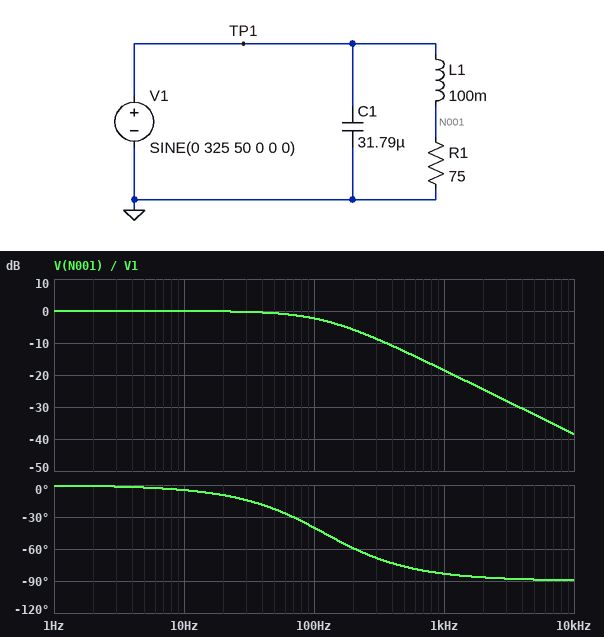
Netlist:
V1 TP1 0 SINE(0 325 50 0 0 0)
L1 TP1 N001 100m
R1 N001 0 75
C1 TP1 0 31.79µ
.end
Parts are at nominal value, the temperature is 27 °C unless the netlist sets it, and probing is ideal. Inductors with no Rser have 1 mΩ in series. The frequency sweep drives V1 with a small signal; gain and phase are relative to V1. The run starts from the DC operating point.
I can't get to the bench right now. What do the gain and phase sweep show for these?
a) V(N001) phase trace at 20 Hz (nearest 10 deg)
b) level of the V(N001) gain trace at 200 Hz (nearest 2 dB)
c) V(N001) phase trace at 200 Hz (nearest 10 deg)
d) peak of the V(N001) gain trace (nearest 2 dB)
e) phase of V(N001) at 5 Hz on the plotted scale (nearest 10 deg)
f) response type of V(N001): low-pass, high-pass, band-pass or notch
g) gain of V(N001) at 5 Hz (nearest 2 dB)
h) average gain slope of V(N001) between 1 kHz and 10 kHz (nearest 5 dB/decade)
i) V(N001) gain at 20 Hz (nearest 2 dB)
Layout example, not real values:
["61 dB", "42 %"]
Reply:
["-10 deg", "-6 dB", "-60 deg", "0 dB", "0 deg", "low-pass", "0 dB", "-20 dB/decade", "0 dB"]
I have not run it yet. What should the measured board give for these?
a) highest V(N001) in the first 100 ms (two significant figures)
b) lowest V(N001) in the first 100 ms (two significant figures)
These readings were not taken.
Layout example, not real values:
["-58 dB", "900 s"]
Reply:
["300 V", "-300 V"]
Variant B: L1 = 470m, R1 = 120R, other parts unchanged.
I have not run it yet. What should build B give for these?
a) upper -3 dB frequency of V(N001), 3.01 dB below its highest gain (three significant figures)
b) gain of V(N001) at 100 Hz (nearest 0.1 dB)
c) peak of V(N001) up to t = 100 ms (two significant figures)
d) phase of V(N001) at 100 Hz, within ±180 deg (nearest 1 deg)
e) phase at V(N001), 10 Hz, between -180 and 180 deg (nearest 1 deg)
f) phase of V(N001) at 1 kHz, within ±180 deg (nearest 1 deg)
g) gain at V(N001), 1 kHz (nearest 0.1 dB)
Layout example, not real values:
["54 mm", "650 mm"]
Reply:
["40.6 Hz", "-8.5 dB", "230 V", "-68 deg", "-14 deg", "-88 deg", "-27.8 dB"]
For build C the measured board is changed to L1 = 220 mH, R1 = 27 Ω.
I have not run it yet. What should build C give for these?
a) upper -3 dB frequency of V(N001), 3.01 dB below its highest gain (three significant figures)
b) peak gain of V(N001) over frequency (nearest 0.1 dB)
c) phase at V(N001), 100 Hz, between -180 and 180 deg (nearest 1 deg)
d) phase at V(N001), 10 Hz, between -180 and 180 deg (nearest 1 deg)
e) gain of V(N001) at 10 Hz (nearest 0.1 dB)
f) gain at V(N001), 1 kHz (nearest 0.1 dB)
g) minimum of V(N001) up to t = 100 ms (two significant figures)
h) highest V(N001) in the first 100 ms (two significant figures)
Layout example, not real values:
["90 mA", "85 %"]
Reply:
["19.5 Hz", "0 dB", "-79 deg", "-27 deg", "-1.0 dB", "-34.2 dB", "-120 V", "160 V"]
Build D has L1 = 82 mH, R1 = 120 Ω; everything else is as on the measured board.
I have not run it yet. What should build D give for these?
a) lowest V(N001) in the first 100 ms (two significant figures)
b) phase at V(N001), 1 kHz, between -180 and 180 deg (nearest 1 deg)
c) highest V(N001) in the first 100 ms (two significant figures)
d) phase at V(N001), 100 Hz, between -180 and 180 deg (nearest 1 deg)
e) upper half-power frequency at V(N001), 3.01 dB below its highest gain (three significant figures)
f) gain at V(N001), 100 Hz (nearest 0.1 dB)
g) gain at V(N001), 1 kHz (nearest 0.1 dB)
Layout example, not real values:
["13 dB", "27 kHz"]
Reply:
["-320 V", "-77 deg", "320 V", "-23 deg", "233 Hz", "-0.7 dB", "-12.9 dB"]
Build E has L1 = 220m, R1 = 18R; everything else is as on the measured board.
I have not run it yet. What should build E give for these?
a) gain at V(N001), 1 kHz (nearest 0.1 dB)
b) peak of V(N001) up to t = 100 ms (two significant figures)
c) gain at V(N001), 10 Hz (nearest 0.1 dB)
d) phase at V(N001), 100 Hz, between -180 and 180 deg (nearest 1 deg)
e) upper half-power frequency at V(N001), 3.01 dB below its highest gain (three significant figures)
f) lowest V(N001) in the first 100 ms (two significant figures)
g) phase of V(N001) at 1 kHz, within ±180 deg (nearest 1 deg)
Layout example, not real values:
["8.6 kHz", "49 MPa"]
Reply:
["-37.7 dB", "120 V", "-2.0 dB", "-83 deg", "13.0 Hz", "-82 V", "-89 deg"]
